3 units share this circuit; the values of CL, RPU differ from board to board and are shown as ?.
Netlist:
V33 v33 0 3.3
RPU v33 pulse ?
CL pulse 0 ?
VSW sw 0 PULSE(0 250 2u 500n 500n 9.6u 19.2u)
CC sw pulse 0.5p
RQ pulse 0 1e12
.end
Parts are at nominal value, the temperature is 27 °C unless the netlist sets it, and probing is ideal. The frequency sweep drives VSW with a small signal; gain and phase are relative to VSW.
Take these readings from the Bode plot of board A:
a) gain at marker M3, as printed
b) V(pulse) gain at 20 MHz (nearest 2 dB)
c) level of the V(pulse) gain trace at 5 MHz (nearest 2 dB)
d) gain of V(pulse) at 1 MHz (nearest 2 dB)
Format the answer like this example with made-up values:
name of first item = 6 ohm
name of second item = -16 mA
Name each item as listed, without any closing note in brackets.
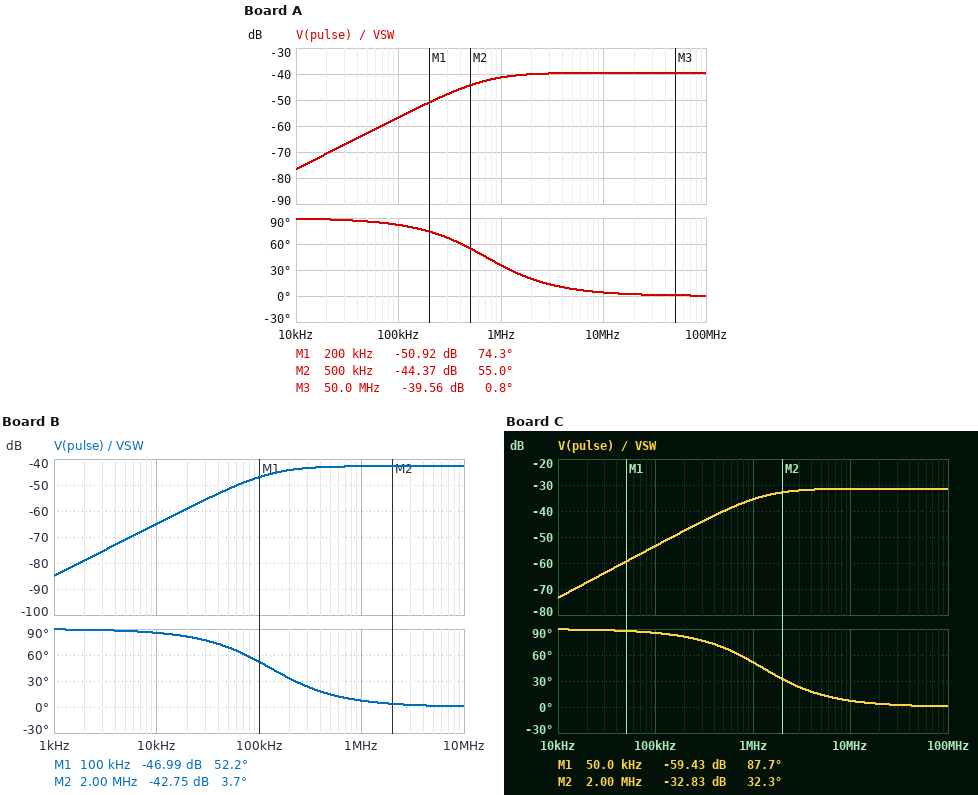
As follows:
gain at marker M3, as printed = -39.56 dB
V(pulse) gain at 20 MHz = -40 dB
level of the V(pulse) gain trace at 5 MHz = -40 dB
gain of V(pulse) at 1 MHz = -42 dB
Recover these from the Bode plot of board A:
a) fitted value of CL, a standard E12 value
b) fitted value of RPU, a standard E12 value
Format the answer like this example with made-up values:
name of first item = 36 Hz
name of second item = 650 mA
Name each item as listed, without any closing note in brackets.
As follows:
fitted value of CL, a standard E12 value = 47 pF
fitted value of RPU, a standard E12 value = 4.7 kΩ
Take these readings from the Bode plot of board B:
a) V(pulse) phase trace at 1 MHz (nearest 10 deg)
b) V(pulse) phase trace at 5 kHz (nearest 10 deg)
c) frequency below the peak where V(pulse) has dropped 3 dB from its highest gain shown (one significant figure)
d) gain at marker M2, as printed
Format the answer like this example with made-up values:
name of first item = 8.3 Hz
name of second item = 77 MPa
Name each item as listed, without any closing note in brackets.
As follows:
V(pulse) phase trace at 1 MHz = 10 deg
V(pulse) phase trace at 5 kHz = 90 deg
frequency below the peak where V(pulse) has dropped 3 dB from its highest gain shown = 100 kHz
gain at marker M2, as printed = -42.75 dB
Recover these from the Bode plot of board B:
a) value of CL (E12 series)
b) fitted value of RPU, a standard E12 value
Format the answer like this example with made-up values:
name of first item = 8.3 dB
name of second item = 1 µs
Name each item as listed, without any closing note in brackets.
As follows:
value of CL = 68 pF
fitted value of RPU, a standard E12 value = 18 kΩ
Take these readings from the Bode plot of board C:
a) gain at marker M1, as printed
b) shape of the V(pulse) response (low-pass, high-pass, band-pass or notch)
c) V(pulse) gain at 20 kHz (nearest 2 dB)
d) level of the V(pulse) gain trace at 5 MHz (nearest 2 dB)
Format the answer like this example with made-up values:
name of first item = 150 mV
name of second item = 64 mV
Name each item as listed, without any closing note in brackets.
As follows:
gain at marker M1, as printed = -59.43 dB
shape of the V(pulse) response = high-pass
V(pulse) gain at 20 kHz = -68 dB
level of the V(pulse) gain trace at 5 MHz = -32 dB
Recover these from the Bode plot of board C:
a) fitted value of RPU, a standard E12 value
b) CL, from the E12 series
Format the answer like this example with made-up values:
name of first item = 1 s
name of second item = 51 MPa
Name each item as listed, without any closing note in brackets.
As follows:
fitted value of RPU, a standard E12 value = 6.8 kΩ
CL, from the E12 series = 18 pF
